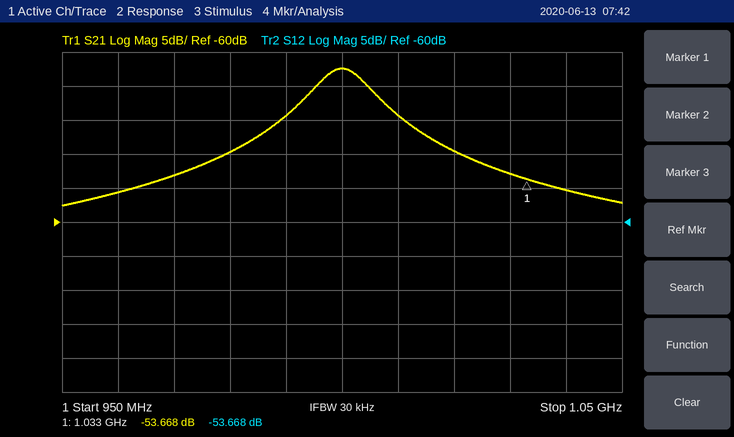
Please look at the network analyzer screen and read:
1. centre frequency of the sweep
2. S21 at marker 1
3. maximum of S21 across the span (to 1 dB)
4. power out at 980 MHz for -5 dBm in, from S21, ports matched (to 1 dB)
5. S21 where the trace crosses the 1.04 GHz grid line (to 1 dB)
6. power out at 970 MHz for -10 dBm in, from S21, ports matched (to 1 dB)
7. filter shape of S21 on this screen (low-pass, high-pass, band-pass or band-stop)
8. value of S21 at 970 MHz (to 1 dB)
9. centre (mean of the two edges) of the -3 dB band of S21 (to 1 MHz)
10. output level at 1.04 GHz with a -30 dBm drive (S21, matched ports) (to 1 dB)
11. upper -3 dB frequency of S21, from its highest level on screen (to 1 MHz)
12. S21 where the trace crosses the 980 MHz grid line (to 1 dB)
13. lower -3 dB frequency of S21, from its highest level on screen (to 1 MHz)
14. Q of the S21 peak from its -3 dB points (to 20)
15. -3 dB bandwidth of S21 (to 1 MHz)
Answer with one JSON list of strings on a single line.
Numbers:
["1 GHz", "-53.668 dB", "-37 dB", "-55 dBm", "-55 dB", "-63 dBm", "band-pass", "-53 dB", "1.000 GHz", "-85 dBm", "1.005 GHz", "-50 dB", "995 MHz", "100", "10 MHz"]
